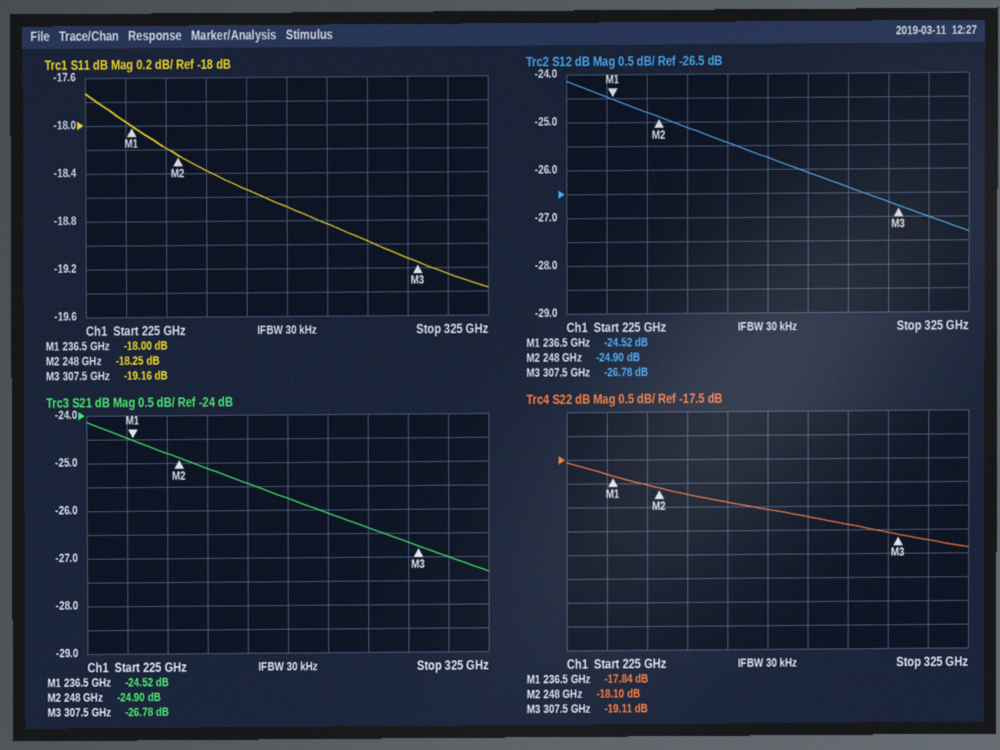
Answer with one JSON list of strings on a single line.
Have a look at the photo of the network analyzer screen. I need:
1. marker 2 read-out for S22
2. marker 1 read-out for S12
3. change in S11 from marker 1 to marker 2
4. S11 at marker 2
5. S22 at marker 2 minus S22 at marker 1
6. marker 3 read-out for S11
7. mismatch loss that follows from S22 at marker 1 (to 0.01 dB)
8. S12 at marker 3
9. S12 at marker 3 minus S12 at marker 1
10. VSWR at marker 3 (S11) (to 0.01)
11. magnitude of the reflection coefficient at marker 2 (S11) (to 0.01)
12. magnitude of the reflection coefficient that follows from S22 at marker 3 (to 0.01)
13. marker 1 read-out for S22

["-18.10 dB", "-24.52 dB", "-0.25 dB", "-18.25 dB", "-0.26 dB", "-19.16 dB", "0.07 dB", "-26.78 dB", "-2.26 dB", "1.25", "0.12", "0.11", "-17.84 dB"]
